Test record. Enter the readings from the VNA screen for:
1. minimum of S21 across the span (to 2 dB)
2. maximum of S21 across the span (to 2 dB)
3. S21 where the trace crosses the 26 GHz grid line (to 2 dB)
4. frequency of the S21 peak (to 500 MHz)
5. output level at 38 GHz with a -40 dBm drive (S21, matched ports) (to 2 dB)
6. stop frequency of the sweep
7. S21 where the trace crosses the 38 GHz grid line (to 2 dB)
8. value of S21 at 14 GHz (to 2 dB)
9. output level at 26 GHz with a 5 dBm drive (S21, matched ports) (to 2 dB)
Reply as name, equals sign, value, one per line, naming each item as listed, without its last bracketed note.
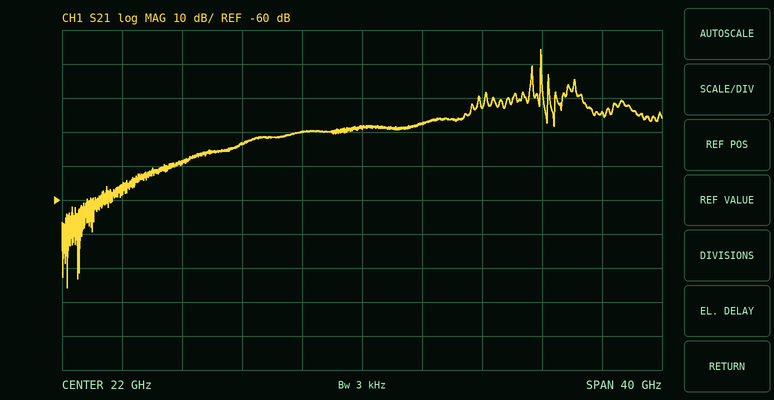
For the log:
minimum of S21 across the span = -86 dB
maximum of S21 across the span = -16 dB
S21 where the trace crosses the 26 GHz grid line = -38 dB
frequency of the S21 peak = 34.0 GHz
output level at 38 GHz with a -40 dBm drive (S21, matched ports) = -74 dBm
stop frequency of the sweep = 42 GHz
S21 where the trace crosses the 38 GHz grid line = -34 dB
value of S21 at 14 GHz = -44 dB
output level at 26 GHz with a 5 dBm drive (S21, matched ports) = -32 dBm
